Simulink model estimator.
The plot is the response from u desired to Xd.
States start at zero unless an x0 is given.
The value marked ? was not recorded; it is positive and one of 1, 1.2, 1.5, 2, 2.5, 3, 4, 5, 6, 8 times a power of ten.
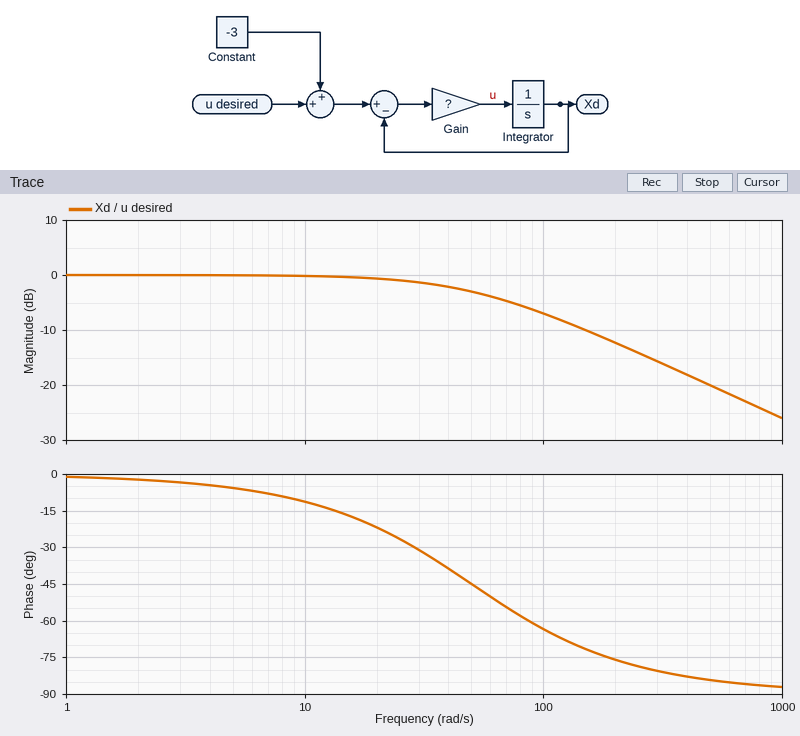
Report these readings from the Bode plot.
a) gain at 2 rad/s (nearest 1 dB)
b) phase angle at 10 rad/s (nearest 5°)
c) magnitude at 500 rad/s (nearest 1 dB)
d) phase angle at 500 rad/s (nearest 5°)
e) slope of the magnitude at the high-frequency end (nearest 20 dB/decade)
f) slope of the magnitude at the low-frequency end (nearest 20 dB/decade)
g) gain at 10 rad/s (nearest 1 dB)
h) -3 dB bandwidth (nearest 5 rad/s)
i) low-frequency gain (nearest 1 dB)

0 dB
-10°
-20 dB
-85°
-20 dB/decade
0 dB/decade
0 dB
50 rad/s
0 dB
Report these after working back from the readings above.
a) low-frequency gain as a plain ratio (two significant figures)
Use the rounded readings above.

1.0
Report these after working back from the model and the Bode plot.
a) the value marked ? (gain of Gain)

50
